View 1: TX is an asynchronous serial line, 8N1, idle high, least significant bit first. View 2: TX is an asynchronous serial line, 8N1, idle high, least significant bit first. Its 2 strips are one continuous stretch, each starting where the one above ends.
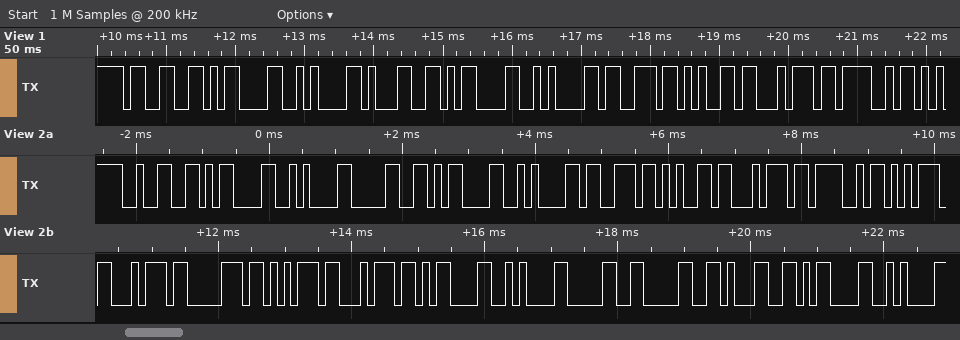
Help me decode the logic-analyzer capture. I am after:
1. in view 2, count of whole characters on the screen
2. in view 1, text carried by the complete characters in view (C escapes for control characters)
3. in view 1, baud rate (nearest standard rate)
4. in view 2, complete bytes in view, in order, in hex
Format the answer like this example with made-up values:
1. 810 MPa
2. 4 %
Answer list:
1. 22
2. "3\r\n1\r\nsetO"
3. 9600 baud
4. 32 0D 0A 30 0D 0A 73 65 74 4F 75 74 70 75 74 0D 0A 30 30 31 0D 0A
